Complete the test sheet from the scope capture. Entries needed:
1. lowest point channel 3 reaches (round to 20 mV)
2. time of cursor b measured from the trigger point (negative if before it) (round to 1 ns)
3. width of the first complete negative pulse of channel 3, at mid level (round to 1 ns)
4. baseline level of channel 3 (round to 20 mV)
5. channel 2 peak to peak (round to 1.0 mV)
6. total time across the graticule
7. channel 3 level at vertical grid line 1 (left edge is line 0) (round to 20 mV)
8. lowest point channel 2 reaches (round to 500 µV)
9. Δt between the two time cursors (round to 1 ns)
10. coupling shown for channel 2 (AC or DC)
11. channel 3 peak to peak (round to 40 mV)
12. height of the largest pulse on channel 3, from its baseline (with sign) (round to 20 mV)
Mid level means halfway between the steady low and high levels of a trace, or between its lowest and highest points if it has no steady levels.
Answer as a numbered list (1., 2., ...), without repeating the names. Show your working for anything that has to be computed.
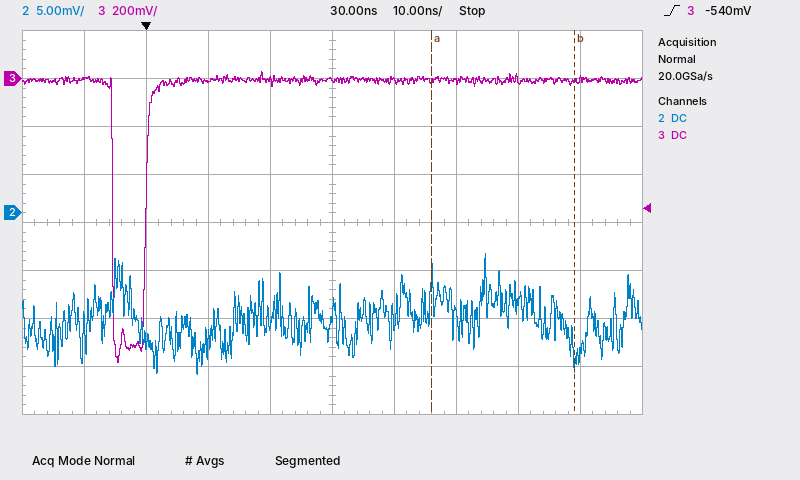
1. -1.18 V
2. +69 ns
3. 5 ns
4. 0 mV
5. 13.0 mV
6. 100 ns
7. 0 mV
8. -17.0 mV
9. 23 ns
10. DC
11. 1.20 V
12. -1.18 V − (0 mV) = -1.18 V
